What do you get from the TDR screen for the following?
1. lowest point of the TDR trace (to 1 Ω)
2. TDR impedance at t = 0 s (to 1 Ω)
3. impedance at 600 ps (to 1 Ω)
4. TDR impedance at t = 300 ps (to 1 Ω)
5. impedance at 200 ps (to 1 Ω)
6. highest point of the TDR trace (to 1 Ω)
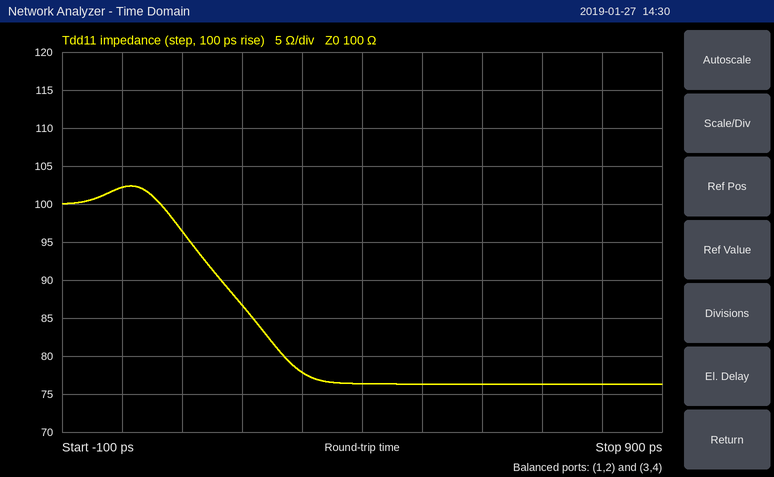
76 Ω
102 Ω
76 Ω
78 Ω
87 Ω
102 Ω
